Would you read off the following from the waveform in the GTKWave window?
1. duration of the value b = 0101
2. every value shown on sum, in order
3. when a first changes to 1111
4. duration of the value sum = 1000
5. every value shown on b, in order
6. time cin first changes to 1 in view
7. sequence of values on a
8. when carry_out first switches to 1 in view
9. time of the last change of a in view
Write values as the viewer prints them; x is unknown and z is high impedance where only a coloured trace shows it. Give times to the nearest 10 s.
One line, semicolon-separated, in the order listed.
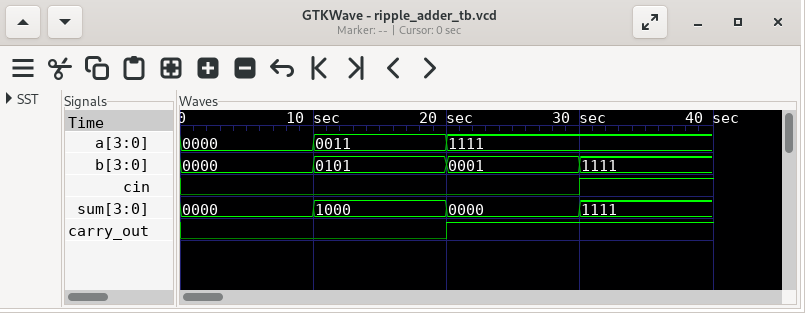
10 s; 0000, 1000, 0000, 1111; 20 s; 10 s; 0000, 0101, 0001, 1111; 30 s; 0000, 0011, 1111; 20 s; 20 s
